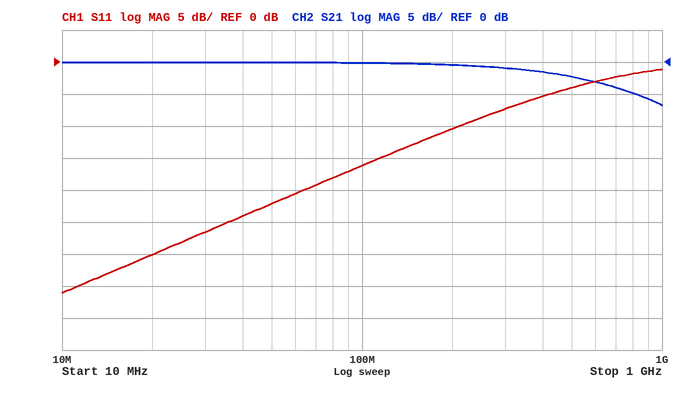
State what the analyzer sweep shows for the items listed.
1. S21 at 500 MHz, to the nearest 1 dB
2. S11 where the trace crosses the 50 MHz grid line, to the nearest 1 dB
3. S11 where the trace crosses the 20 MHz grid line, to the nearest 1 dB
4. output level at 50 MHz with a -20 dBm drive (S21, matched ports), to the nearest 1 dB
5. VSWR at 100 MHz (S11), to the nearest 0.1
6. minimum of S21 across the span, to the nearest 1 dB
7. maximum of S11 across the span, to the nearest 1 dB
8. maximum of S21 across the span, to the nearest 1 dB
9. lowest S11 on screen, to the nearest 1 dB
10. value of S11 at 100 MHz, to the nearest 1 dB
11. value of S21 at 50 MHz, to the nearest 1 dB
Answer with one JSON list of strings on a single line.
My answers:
["-2 dB", "-22 dB", "-30 dB", "-20 dBm", "1.4", "-7 dB", "-1 dB", "0 dB", "-36 dB", "-16 dB", "0 dB"]
